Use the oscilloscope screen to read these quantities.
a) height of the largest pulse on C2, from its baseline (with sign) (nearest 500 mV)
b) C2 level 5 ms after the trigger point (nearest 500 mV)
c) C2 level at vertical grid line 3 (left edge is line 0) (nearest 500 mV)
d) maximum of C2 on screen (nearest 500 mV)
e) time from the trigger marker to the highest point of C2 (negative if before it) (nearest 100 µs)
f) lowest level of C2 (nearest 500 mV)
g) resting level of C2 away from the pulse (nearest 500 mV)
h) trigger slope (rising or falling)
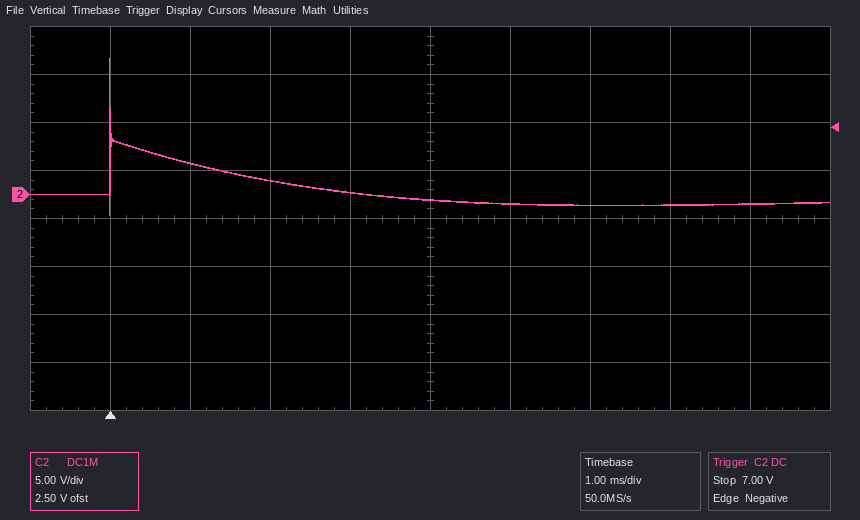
+15.0 V
-1.0 V
1.5 V
14.0 V
0.0 ms
-2.0 V
-1.0 V
falling
